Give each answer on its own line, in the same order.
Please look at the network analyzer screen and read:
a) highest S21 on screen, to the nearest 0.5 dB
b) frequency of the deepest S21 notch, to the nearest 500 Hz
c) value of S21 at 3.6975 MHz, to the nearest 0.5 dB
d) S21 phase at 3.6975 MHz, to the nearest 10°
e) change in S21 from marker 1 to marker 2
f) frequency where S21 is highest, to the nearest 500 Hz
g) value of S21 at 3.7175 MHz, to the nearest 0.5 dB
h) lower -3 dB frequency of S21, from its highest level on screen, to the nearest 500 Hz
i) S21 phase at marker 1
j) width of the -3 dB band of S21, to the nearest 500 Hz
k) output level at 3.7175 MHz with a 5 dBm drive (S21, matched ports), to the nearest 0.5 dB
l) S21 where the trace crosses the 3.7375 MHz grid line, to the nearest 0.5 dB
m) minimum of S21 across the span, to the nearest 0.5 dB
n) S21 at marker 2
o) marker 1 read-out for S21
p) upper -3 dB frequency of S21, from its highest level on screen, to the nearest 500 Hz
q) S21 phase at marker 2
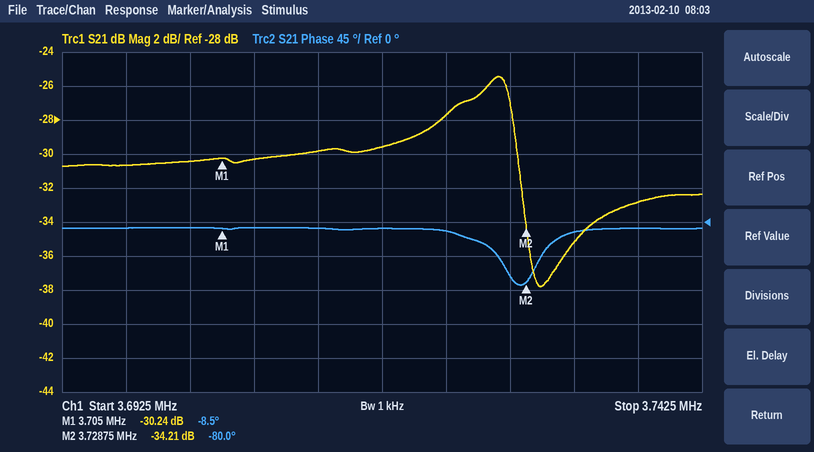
-25.5 dB
3.7300 MHz
-30.5 dB
-10°
-3.97 dB
3.7265 MHz
-29.5 dB
3.7215 MHz
-8.5°
6.5 kHz
-24.5 dBm
-33.0 dB
-38.0 dB
-34.21 dB
-30.24 dB
3.7280 MHz
-80.0°
